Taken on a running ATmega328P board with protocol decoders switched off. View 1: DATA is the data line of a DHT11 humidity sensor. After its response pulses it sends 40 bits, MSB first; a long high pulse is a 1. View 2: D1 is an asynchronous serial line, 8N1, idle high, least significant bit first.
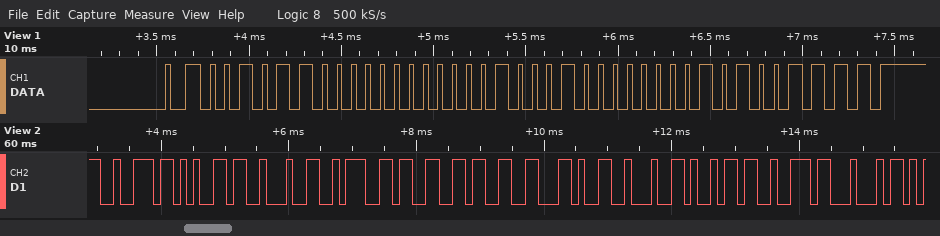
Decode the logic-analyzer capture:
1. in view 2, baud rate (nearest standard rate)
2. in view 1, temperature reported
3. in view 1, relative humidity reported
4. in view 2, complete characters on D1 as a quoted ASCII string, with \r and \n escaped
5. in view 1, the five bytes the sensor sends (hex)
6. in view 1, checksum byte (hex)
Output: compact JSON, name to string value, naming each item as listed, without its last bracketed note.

{"in view 2, baud rate": "9600 baud", "in view 1, temperature reported": "34.1 °C", "in view 1, relative humidity reported": "44 %", "in view 2, complete characters on D1 as a quoted ASCII string, with \\r and \\n escaped": "\"re\\\":33,\\\"irD\"", "in view 1, the five bytes the sensor sends": "2C 00 22 01 4F", "in view 1, checksum byte": "0x4F"}
